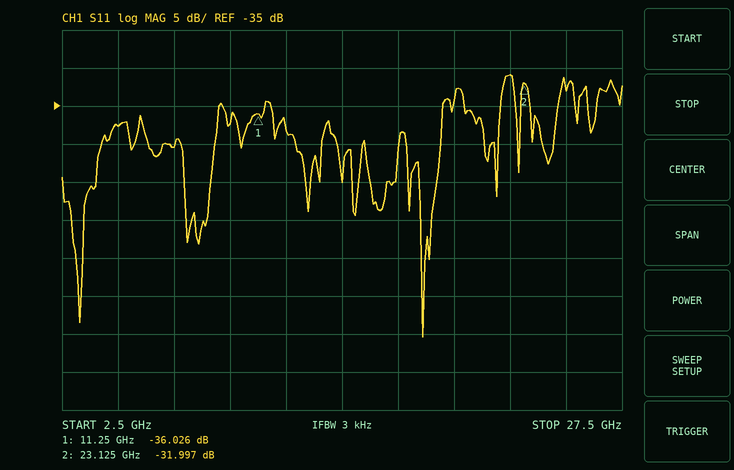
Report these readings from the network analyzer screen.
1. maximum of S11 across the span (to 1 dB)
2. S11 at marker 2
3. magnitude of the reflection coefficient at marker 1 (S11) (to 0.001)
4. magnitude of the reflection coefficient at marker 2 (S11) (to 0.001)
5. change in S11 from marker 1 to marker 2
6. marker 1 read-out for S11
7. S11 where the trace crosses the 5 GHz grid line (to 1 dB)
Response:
-31 dB
-31.997 dB
0.016
0.025
4.029 dB
-36.026 dB
-38 dB
